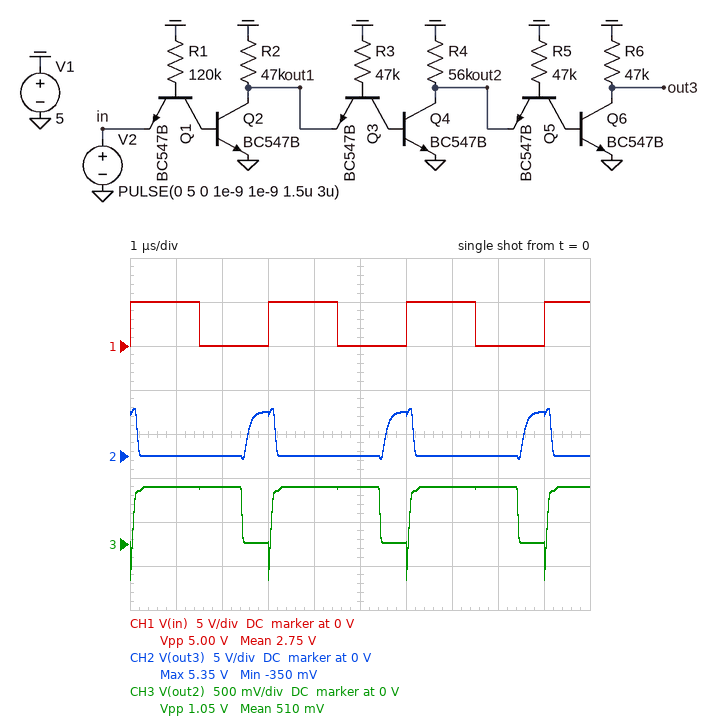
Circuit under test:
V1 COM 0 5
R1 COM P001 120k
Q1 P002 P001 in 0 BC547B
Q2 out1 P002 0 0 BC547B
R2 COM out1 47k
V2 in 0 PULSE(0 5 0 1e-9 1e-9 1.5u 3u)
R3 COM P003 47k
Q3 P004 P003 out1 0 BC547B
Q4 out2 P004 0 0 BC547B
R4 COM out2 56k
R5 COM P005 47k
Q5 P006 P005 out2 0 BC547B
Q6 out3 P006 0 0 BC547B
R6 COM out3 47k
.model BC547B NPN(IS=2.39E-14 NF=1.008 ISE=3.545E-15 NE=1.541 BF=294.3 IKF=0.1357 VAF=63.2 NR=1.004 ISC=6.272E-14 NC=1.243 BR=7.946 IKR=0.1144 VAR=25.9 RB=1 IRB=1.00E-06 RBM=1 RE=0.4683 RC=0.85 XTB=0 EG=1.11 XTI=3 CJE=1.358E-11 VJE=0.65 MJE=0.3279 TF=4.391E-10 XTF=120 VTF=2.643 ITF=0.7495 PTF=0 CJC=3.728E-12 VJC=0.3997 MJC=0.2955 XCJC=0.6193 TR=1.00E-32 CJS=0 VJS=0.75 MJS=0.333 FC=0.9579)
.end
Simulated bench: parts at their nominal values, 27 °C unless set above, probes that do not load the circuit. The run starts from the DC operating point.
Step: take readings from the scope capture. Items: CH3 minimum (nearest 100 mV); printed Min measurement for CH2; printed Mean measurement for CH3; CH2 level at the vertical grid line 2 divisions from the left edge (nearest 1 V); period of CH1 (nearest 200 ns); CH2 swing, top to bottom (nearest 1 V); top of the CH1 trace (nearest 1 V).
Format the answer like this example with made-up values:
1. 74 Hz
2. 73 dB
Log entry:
1. -400 mV
2. -350 mV
3. 510 mV
4. 0 V
5. 3.0 µs
6. 6 V
7. 5 V
